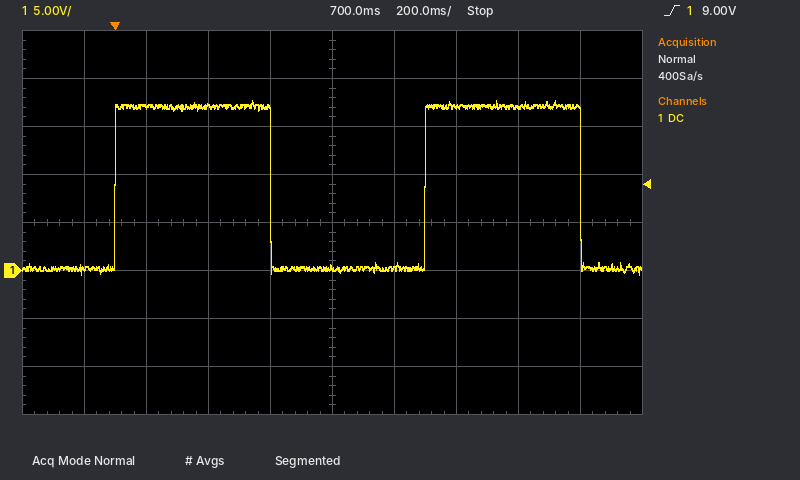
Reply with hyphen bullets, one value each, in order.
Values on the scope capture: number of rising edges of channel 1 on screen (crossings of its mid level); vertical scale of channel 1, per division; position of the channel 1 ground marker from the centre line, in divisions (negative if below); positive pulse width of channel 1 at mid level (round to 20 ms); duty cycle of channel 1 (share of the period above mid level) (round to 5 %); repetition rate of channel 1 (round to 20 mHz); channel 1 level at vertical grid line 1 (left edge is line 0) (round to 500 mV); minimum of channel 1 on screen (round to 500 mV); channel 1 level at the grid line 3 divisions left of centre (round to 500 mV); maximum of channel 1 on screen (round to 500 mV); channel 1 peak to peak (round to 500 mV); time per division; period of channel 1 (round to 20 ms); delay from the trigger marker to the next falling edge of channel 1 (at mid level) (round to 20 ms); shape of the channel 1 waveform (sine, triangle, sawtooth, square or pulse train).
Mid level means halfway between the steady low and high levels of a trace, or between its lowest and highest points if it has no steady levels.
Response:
- 2
- 5 V
- -1.0 div
- 500 ms
- 50 %
- 1.00 Hz
- 0.0 V
- -500 mV
- 17.0 V
- 17.5 V
- 18.0 V
- 200 ms
- 1.00 s
- 500 ms
- square
